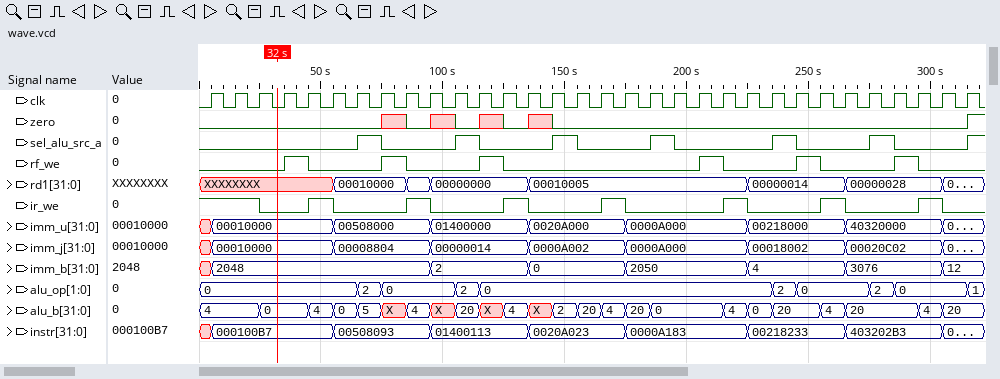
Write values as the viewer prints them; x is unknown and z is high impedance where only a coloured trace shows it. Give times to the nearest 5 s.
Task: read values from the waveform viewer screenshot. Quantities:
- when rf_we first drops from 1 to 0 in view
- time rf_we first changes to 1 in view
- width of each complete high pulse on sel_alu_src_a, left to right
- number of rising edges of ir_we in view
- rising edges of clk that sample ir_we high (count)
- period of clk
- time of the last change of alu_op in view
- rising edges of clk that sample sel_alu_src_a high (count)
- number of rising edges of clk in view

45 s
35 s
10 s, 10 s, 10 s, 10 s, 10 s, 10 s
7
10
10 s
315 s
6
32
